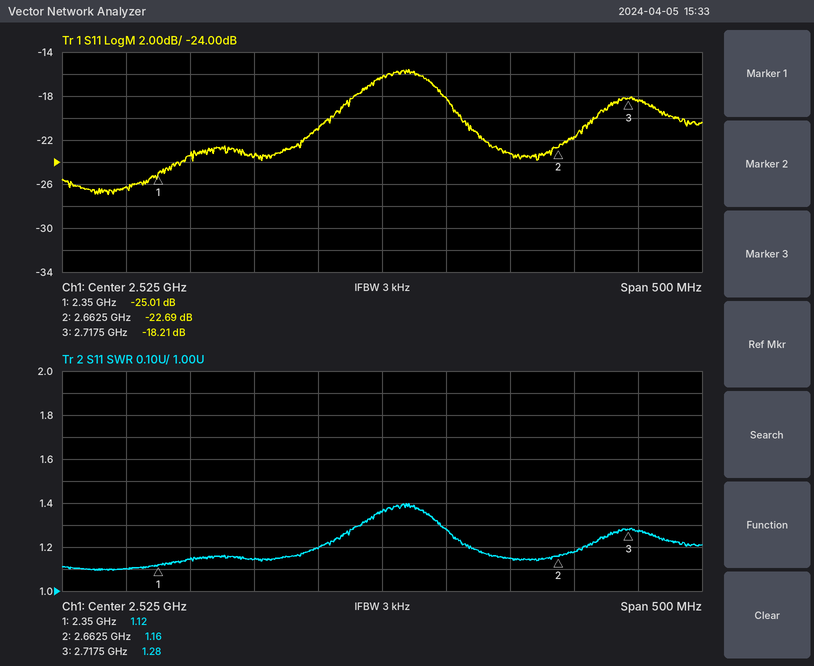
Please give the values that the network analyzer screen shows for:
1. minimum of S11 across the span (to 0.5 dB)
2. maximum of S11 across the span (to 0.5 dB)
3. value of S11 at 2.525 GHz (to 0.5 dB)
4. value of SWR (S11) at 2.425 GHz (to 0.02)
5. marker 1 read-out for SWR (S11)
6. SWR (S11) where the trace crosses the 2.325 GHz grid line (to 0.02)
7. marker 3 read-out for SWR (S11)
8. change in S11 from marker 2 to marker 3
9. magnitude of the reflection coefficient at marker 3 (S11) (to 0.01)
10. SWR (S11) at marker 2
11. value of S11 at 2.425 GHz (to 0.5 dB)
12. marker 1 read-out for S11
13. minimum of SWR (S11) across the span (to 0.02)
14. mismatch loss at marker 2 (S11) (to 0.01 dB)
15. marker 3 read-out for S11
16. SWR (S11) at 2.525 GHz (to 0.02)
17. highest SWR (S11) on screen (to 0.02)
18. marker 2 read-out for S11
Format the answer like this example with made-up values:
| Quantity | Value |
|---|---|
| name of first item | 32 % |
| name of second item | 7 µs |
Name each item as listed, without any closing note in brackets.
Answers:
| Quantity | Value |
|---|---|
| minimum of S11 across the span | -27.0 dB |
| maximum of S11 across the span | -15.5 dB |
| value of S11 at 2.525 GHz | -16.5 dB |
| value of SWR (S11) at 2.425 GHz | 1.14 |
| marker 1 read-out for SWR | 1.12 |
| SWR (S11) where the trace crosses the 2.325 GHz grid line | 1.10 |
| marker 3 read-out for SWR | 1.28 |
| change in S11 from marker 2 to marker 3 | 4.48 dB |
| magnitude of the reflection coefficient at marker 3 (S11) | 0.12 |
| SWR (S11) at marker 2 | 1.16 |
| value of S11 at 2.425 GHz | -23.5 dB |
| marker 1 read-out for S11 | -25.01 dB |
| minimum of SWR (S11) across the span | 1.10 |
| mismatch loss at marker 2 (S11) | 0.02 dB |
| marker 3 read-out for S11 | -18.21 dB |
| SWR (S11) at 2.525 GHz | 1.36 |
| highest SWR (S11) on screen | 1.40 |
| marker 2 read-out for S11 | -22.69 dB |
